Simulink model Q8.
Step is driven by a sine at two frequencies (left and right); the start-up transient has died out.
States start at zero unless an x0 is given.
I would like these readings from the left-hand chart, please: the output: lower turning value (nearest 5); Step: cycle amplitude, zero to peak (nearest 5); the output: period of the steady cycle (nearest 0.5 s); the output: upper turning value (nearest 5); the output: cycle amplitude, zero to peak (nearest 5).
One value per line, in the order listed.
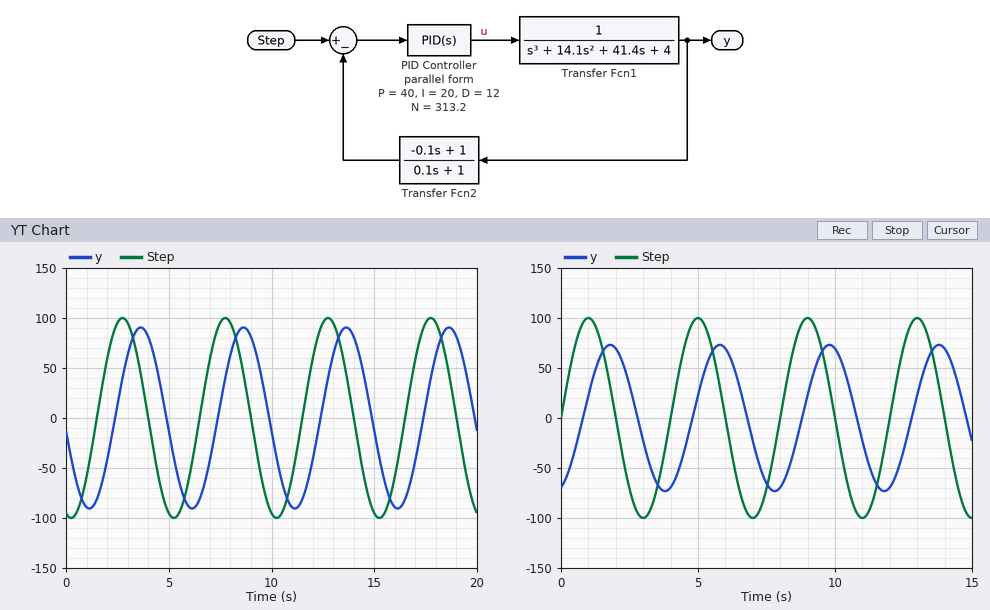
-90
100
5.0 s
90
90
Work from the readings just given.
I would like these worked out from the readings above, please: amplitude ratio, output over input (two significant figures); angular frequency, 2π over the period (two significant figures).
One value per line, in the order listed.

0.90
1.3 rad/s
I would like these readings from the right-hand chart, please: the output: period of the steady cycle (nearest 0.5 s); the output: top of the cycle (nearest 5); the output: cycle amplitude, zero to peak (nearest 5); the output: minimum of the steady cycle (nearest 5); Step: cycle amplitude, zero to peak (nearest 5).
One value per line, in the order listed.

4.0 s
75
75
-75
100
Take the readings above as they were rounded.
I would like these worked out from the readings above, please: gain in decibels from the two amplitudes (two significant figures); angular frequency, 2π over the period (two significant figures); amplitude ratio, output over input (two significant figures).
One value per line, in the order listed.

-2.5 dB
1.6 rad/s
0.75
